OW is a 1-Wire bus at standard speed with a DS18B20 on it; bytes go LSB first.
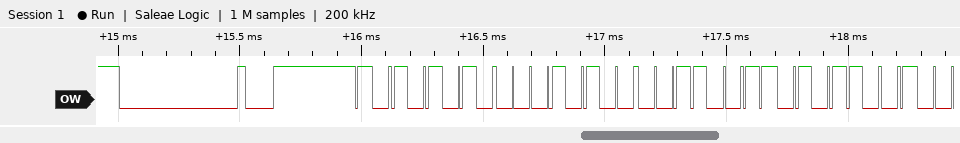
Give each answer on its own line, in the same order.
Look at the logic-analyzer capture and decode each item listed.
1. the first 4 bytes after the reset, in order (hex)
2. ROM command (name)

55 28 CC 9A
Match ROM
